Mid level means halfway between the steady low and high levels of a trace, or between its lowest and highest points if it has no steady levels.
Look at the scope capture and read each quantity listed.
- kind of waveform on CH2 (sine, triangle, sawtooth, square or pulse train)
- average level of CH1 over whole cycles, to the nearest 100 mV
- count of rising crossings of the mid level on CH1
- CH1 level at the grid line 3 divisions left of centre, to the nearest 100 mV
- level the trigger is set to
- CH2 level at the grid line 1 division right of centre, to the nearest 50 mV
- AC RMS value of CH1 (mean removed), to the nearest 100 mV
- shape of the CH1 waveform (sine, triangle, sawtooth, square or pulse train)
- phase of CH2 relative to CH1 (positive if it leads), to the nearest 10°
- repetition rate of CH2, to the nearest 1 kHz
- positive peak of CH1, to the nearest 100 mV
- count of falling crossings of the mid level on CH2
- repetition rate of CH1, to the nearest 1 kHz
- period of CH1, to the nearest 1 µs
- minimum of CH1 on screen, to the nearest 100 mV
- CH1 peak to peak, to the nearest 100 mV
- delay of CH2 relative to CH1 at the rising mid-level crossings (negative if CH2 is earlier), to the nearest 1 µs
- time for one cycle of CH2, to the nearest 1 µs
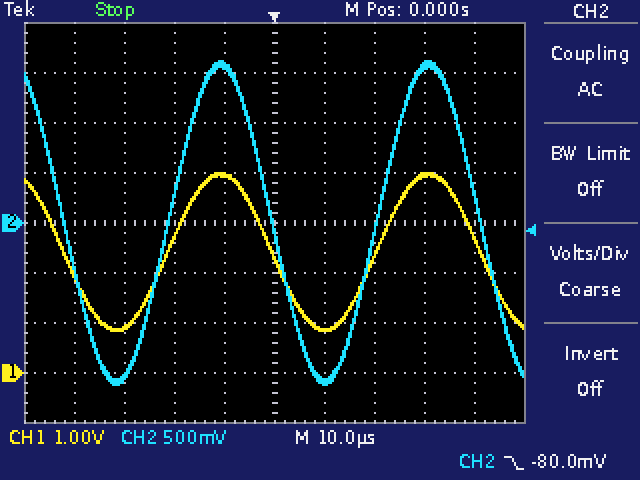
sine
2.4 V
2
900 mV
-80.0 mV
-1.60 V
1.1 V
sine
0°
24 kHz
4.0 V
3
24 kHz
42 µs
800 mV
3.2 V
0 µs
42 µs
